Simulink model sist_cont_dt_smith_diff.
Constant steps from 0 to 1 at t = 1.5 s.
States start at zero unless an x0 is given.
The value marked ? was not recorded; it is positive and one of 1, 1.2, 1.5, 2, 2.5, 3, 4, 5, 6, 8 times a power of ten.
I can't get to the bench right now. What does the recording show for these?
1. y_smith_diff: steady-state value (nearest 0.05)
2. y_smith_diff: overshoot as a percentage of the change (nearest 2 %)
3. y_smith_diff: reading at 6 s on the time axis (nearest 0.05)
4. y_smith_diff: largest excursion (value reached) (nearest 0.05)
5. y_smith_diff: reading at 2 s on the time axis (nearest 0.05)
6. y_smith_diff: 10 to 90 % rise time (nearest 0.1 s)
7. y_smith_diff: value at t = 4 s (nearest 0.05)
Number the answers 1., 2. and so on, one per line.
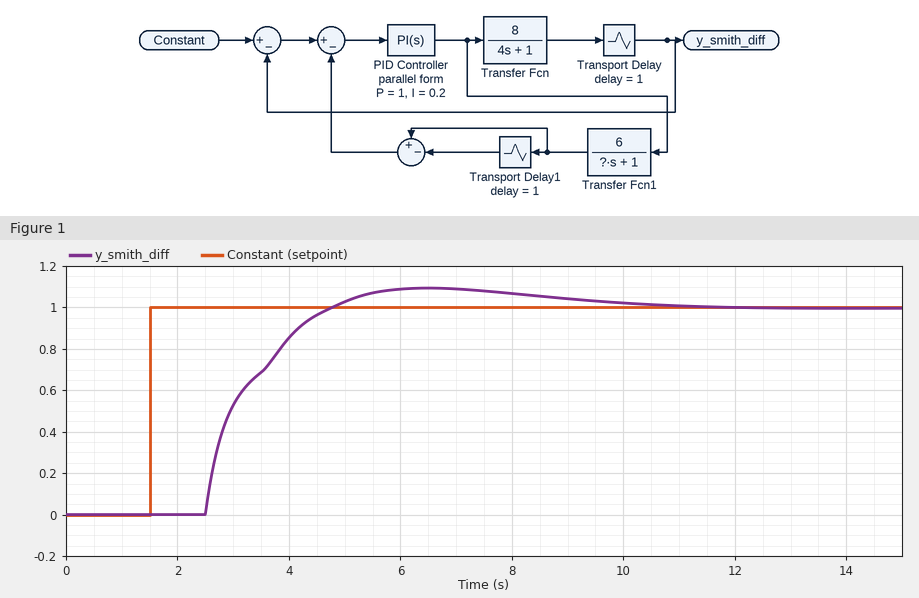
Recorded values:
1. 1.00
2. 10 %
3. 1.10
4. 1.10
5. 0.00
6. 1.6 s
7. 0.85
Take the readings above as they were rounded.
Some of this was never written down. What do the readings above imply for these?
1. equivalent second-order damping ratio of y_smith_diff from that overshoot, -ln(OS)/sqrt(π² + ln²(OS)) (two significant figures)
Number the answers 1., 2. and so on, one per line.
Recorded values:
1. 0.59
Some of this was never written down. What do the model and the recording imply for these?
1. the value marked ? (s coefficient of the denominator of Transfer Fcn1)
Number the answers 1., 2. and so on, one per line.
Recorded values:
1. 2
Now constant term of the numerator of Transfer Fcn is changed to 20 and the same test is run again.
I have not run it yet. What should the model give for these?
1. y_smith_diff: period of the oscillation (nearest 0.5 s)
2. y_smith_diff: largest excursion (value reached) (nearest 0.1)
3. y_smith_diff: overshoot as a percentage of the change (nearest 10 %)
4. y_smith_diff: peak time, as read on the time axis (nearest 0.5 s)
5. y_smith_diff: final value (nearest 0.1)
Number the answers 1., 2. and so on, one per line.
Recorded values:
1. 3.0 s
2. 1.7
3. 70 %
4. 3.5 s
5. 1.0
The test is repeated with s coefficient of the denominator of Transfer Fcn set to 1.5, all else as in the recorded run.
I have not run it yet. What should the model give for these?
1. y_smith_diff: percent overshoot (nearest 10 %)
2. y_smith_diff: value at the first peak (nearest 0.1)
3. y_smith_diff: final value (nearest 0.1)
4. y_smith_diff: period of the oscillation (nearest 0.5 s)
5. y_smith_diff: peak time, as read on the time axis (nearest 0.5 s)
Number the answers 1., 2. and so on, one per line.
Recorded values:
1. 40 %
2. 1.4
3. 1.0
4. 2.5 s
5. 3.5 s
